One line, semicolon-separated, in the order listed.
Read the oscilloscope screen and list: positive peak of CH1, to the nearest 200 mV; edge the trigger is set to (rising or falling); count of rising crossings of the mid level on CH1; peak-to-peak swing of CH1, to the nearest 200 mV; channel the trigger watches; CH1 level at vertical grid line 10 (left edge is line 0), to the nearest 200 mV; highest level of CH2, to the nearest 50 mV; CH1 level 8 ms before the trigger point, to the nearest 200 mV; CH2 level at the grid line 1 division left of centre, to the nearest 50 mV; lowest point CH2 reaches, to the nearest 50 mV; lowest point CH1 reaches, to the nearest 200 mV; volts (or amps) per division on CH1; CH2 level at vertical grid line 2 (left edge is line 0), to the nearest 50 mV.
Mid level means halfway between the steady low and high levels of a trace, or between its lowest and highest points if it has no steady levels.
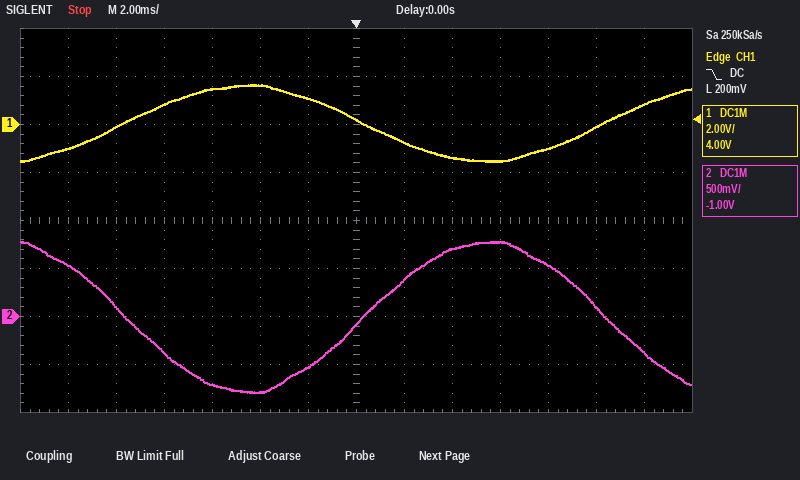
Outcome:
1.6 V; falling; 2; 3.2 V; CH1; -1.6 V; 800 mV; 800 mV; -550 mV; -800 mV; -1.6 V; 2 V; 100 mV
